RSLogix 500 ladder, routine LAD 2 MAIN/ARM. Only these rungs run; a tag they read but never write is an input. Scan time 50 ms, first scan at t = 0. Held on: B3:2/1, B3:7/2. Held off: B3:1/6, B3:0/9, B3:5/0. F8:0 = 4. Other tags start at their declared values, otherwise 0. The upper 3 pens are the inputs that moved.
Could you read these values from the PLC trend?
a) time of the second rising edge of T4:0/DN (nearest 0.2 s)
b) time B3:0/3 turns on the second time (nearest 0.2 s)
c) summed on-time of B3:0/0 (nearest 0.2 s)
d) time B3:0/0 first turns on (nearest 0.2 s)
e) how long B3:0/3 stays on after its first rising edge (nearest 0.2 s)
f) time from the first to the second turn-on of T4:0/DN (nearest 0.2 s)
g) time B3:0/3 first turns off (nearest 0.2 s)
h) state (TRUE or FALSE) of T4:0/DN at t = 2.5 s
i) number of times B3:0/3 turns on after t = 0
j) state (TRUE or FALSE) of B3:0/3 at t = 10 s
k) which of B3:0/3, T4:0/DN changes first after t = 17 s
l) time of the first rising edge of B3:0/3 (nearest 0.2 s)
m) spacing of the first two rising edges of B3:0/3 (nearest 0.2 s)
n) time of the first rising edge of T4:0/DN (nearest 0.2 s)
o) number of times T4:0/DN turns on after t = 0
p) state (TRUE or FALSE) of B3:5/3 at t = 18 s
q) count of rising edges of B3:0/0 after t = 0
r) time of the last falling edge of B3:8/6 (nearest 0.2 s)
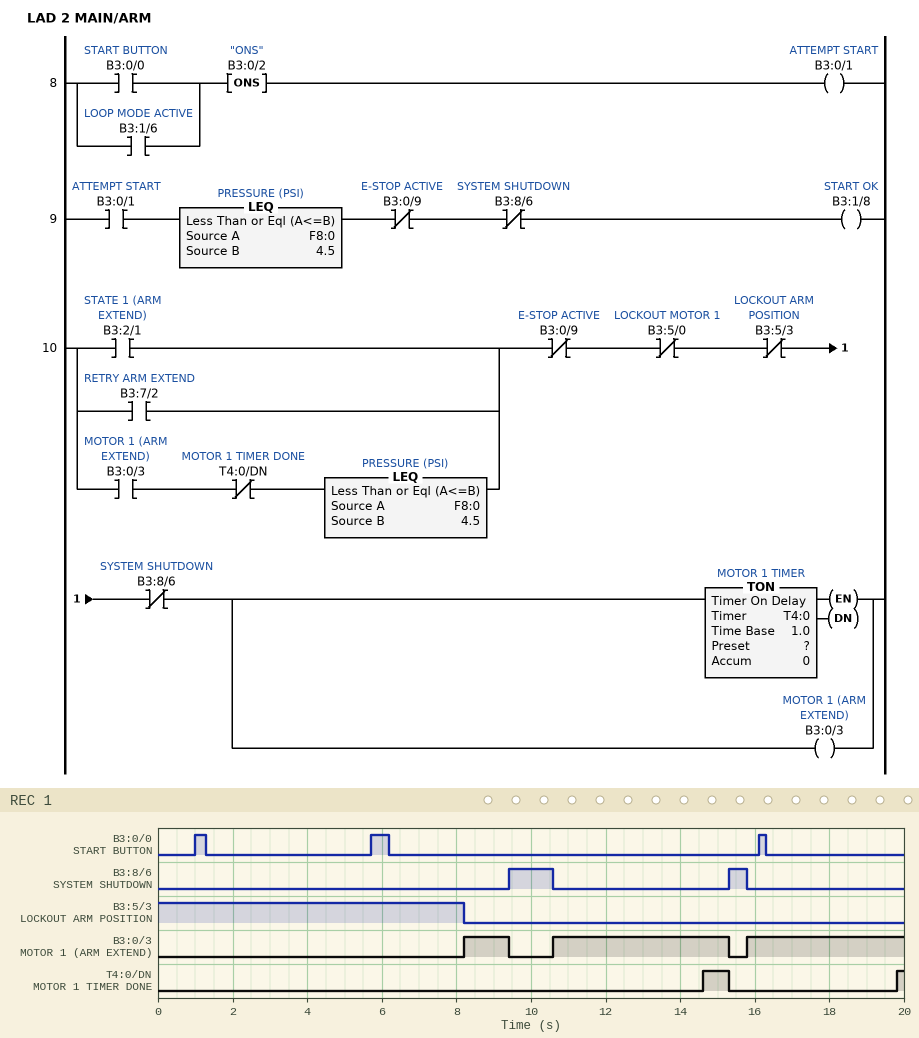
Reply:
19.8 s
10.6 s
1.0 s
1.0 s
1.2 s
5.2 s
9.4 s
FALSE
3
FALSE
T4:0/DN
8.2 s
2.4 s
14.6 s
2
FALSE
3
15.8 s
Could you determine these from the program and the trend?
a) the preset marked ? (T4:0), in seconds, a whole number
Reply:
4 s
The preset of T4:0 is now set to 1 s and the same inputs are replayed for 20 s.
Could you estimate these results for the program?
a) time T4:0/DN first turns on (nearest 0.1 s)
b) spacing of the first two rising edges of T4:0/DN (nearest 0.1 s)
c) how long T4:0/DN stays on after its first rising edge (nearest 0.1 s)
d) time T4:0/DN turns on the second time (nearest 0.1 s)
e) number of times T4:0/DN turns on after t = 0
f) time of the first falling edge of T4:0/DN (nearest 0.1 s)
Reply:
9.2 s
2.4 s
0.2 s
11.6 s
3
9.4 s
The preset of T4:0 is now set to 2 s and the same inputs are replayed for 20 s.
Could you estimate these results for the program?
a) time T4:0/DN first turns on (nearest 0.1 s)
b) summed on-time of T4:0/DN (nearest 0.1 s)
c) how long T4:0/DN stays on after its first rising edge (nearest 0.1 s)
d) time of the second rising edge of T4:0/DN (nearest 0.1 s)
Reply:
12.6 s
4.9 s
2.7 s
17.8 s
